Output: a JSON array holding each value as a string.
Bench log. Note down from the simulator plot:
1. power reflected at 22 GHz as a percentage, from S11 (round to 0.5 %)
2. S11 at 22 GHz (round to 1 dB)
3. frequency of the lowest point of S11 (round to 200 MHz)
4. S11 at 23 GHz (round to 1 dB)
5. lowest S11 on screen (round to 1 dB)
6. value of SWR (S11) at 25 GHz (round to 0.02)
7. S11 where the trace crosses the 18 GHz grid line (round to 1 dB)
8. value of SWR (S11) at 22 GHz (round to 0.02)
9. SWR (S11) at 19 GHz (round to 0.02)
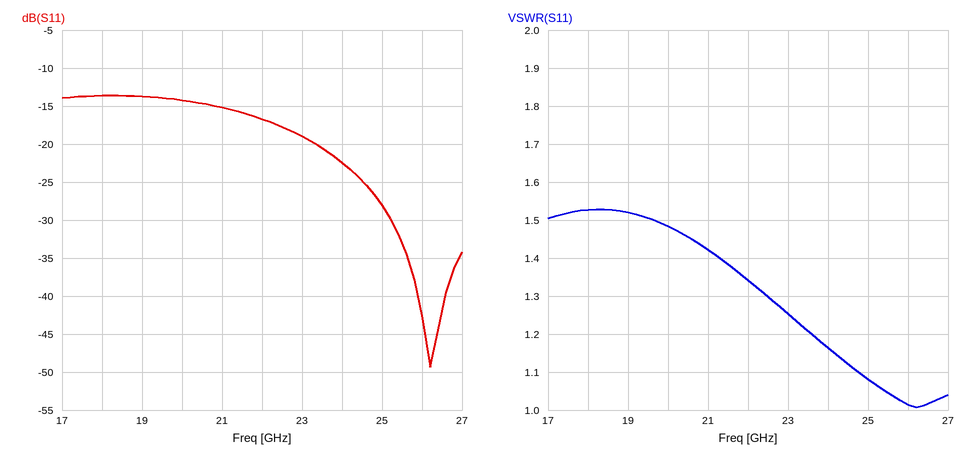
["2.0 %", "-17 dB", "26.2 GHz", "-19 dB", "-49 dB", "1.08", "-14 dB", "1.34", "1.52"]
